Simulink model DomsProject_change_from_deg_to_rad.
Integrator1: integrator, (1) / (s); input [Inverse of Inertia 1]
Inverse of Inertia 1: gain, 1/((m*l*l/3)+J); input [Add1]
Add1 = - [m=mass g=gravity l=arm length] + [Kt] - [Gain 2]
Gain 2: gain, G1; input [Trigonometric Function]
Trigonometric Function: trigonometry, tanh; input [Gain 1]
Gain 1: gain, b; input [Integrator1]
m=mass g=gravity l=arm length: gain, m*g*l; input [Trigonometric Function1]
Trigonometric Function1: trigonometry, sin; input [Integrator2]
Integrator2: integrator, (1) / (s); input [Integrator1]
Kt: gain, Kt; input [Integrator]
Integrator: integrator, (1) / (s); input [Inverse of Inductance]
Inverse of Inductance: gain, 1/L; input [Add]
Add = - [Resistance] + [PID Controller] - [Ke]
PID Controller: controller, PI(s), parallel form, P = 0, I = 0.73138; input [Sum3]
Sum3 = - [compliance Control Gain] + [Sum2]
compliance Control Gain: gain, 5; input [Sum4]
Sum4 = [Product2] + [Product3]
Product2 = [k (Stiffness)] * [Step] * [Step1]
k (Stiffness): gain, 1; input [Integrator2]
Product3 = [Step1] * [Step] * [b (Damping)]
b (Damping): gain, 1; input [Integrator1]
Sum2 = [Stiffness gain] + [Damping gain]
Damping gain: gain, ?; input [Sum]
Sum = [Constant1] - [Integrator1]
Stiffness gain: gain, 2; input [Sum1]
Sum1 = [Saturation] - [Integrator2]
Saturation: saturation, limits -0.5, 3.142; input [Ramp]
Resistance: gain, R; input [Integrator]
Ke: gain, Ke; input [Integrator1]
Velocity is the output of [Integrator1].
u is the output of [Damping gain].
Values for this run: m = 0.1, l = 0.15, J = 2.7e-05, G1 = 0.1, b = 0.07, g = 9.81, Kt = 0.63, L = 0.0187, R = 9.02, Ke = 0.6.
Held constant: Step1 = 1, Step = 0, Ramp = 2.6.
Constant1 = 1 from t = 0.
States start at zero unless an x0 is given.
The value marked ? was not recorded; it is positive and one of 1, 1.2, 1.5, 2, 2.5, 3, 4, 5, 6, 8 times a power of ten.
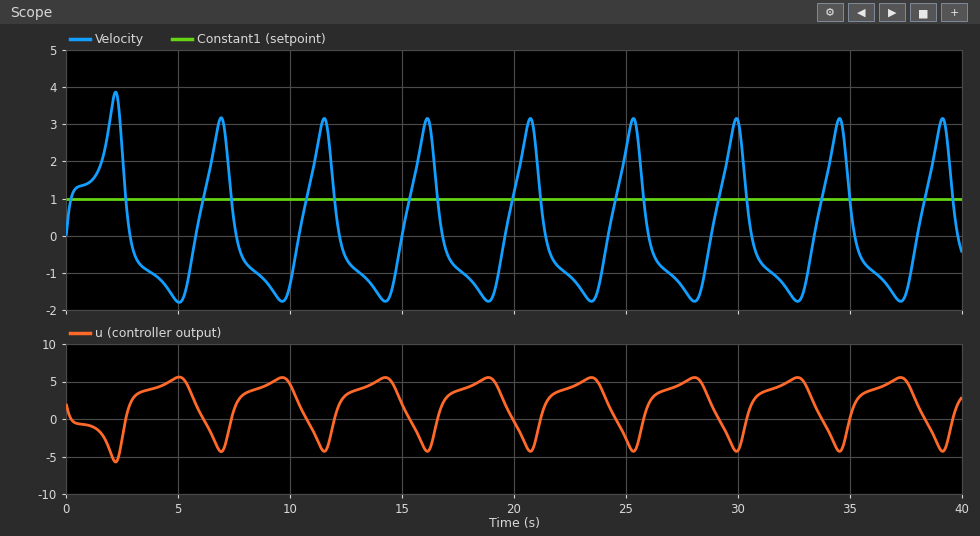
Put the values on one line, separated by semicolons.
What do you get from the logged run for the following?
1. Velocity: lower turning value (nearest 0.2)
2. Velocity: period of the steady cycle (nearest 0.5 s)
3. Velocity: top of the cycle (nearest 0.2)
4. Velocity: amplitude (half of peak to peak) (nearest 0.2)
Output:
-1.8; 4.5 s; 3.2; 2.4
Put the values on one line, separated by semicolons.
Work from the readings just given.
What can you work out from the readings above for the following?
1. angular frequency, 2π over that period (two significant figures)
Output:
1.4 rad/s
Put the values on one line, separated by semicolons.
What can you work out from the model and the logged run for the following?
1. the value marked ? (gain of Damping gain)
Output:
2
